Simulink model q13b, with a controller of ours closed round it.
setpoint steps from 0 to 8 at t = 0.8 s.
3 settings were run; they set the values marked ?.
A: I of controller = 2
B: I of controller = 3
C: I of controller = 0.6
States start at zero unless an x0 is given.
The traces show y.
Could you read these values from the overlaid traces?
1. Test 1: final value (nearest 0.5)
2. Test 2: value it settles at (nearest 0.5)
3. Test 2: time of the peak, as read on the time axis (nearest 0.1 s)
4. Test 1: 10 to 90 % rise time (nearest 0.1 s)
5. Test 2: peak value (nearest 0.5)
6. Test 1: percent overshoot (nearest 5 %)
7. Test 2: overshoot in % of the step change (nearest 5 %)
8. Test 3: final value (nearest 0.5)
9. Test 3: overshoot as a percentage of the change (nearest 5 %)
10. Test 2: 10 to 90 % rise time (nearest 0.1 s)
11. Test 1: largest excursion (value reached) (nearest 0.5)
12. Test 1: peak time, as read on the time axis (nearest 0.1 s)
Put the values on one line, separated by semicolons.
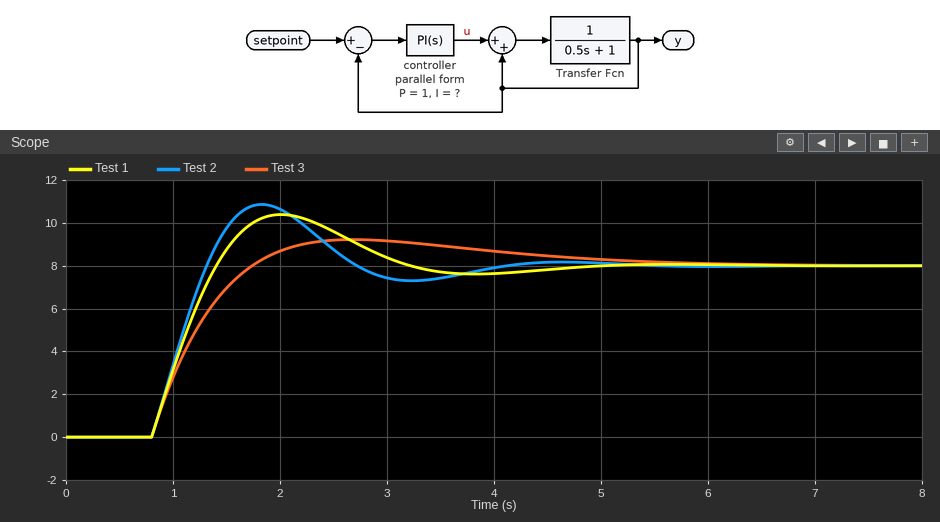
8.0; 8.0; 1.8 s; 0.5 s; 11.0; 30 %; 35 %; 8.0; 15 %; 0.4 s; 10.5; 2.0 s
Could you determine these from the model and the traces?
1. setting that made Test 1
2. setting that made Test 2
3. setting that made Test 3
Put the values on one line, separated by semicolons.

A; B; C
